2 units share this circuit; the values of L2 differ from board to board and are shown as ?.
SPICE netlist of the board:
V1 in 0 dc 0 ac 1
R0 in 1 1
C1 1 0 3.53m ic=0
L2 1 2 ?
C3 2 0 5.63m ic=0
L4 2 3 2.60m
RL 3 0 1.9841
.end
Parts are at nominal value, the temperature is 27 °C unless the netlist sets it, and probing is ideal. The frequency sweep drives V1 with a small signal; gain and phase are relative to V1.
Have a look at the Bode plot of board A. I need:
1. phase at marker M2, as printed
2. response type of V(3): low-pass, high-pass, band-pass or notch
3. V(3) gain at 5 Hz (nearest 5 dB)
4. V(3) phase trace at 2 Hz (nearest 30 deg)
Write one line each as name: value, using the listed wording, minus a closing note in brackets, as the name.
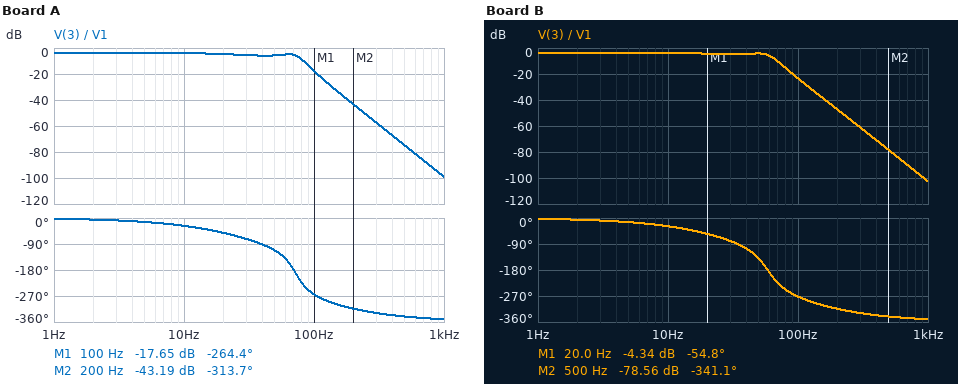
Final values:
phase at marker M2, as printed: -313.7 deg
response type of V(3): low-pass, high-pass, band-pass or notch: low-pass
V(3) gain at 5 Hz: -5 dB
V(3) phase trace at 2 Hz: 0 deg
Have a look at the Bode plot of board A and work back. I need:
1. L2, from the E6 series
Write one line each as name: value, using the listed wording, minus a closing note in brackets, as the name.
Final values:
L2, from the E6 series: 2.2 mH
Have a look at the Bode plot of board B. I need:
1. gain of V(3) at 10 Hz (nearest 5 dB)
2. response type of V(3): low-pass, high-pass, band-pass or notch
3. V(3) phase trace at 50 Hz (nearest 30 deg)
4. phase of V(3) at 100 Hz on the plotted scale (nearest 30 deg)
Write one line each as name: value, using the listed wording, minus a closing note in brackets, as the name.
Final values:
gain of V(3) at 10 Hz: -5 dB
response type of V(3): low-pass, high-pass, band-pass or notch: low-pass
V(3) phase trace at 50 Hz: -150 deg
phase of V(3) at 100 Hz on the plotted scale: -270 deg
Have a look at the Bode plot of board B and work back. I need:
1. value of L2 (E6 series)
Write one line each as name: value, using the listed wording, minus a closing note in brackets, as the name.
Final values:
value of L2: 3.3 mH
